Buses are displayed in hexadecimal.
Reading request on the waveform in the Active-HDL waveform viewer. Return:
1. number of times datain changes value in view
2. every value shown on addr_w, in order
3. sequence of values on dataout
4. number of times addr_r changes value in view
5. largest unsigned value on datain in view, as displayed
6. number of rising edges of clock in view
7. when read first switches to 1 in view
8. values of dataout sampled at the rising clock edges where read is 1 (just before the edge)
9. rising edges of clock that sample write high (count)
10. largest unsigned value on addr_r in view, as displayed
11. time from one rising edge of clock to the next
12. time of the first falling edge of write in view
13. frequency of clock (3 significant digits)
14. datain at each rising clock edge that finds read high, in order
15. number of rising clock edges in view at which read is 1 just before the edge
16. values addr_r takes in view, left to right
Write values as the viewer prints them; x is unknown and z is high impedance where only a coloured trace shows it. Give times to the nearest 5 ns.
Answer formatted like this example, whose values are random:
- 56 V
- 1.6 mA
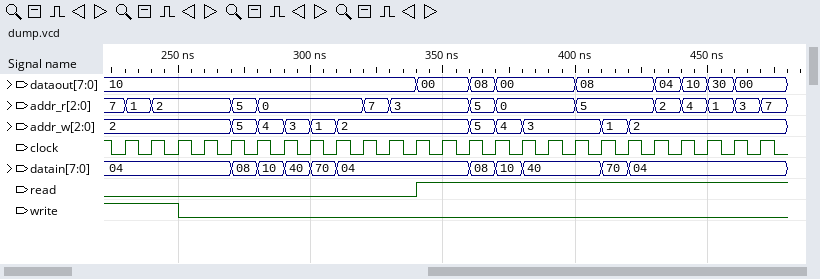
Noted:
- 10
- 2, 5, 4, 3, 1, 2, 5, 4, 3, 1, 2
- 10, 00, 08, 00, 08, 04, 10, 30, 00
- 14
- 70
- 25
- 340 ns
- 00, 00, 08, 00, 00, 00, 08, 08, 08, 04, 10, 30, 00
- 3
- 7
- 10 ns
- 250 ns
- 100 MHz
- 04, 04, 08, 10, 40, 40, 40, 70, 04, 04, 04, 04, 04
- 13
- 7, 1, 2, 5, 0, 7, 3, 5, 0, 5, 2, 4, 1, 3, 7
